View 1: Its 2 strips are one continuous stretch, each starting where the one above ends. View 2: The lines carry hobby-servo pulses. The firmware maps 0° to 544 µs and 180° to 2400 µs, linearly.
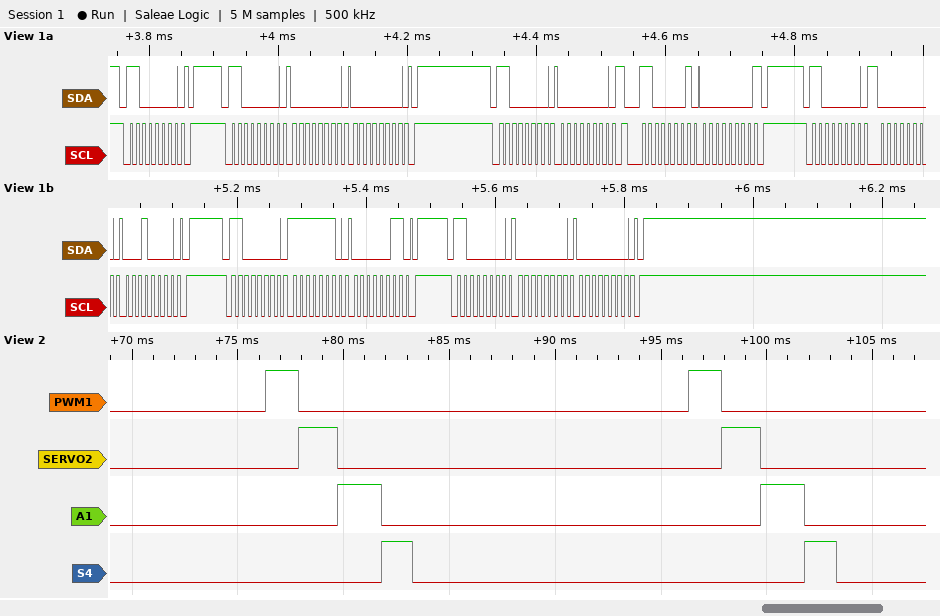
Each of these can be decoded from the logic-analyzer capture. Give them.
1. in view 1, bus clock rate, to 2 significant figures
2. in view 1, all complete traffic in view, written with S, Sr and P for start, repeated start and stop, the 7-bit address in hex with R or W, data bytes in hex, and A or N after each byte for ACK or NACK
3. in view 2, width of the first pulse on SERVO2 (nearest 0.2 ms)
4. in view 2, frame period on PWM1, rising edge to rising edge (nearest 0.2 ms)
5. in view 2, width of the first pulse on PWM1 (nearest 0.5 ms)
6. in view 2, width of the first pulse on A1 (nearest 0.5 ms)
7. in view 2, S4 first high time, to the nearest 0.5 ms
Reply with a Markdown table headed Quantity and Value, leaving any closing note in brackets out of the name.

| Quantity | Value |
|---|---|
| in view 1, bus clock rate, to 2 significant figures | 100 kHz |
| in view 1, all complete traffic in view, written with S, Sr and P for start, repeated start and stop, the 7-bit address in hex with R or W, data bytes in hex, and A or N after each byte for ACK or NACK | S 60W A P S 60W A 00 A 00 A P S 60W A 00 A Sr 60R A 00 N P S 60W A 00 A 10 A P S 60W A FE A 03 A P S 60W A 00 A 00 A P |
| in view 2, width of the first pulse on SERVO2 | 1.8 ms |
| in view 2, frame period on PWM1, rising edge to rising edge | 20.0 ms |
| in view 2, width of the first pulse on PWM1 | 1.5 ms |
| in view 2, width of the first pulse on A1 | 2.0 ms |
| in view 2, S4 first high time, to the nearest 0.5 ms | 1.5 ms |
